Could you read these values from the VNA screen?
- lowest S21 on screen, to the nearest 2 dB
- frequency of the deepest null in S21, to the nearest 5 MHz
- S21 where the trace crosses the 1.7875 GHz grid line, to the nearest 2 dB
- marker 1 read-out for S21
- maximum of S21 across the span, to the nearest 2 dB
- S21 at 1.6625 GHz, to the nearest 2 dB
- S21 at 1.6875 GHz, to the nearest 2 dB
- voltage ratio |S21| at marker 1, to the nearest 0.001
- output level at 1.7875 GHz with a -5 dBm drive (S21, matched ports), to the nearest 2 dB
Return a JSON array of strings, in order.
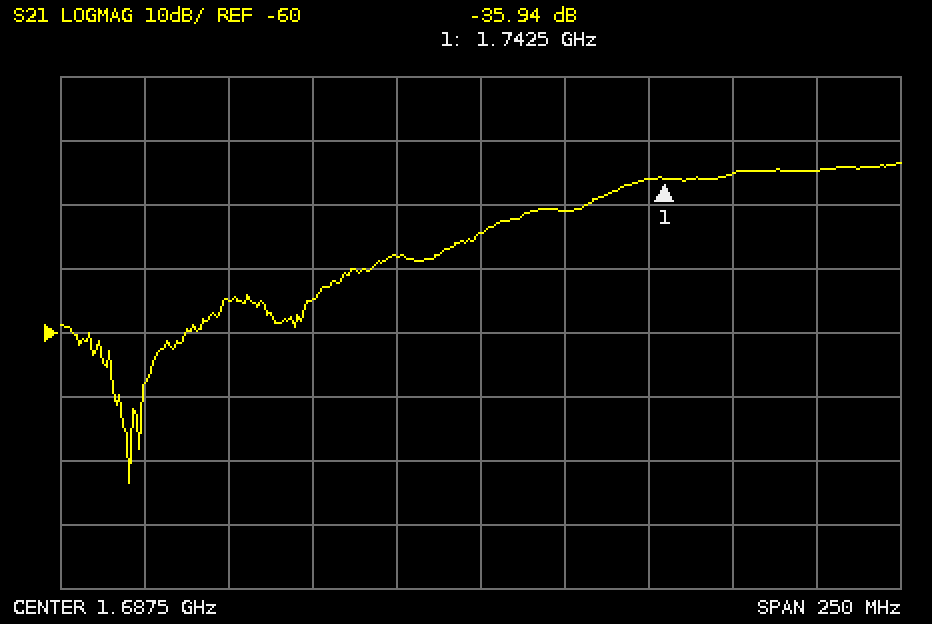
["-84 dB", "1.585 GHz", "-34 dB", "-35.94 dB", "-34 dB", "-48 dB", "-44 dB", "0.016", "-40 dBm"]
